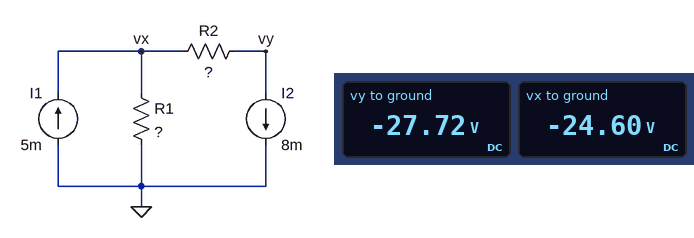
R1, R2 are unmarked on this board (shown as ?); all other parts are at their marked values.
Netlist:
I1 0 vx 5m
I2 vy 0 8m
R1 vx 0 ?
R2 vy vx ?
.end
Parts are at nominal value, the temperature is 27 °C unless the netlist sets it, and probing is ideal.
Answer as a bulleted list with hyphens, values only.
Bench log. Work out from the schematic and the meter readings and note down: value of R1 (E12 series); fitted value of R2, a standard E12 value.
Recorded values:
- 8.2 kΩ
- 390 Ω
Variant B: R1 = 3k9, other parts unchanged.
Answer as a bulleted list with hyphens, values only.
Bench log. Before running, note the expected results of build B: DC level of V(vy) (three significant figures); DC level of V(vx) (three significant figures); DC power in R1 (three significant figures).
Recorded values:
- -14.8 V
- -11.7 V
- 35.1 mW
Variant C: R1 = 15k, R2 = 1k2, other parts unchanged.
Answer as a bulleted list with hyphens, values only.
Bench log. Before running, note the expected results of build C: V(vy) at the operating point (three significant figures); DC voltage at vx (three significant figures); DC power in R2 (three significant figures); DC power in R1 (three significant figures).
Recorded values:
- -54.6 V
- -45.0 V
- 76.8 mW
- 135 mW
